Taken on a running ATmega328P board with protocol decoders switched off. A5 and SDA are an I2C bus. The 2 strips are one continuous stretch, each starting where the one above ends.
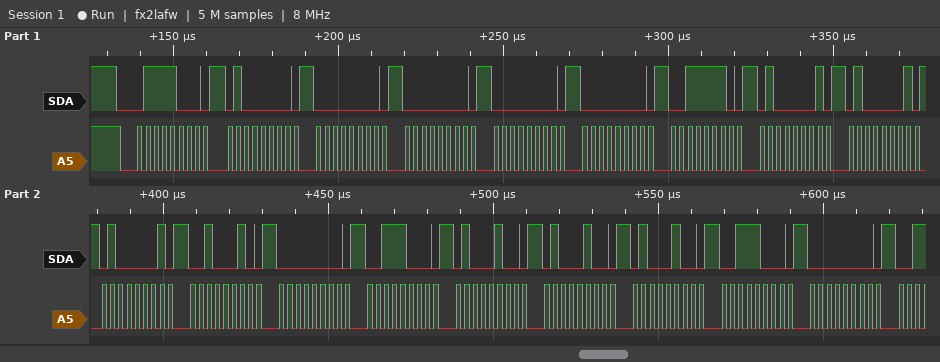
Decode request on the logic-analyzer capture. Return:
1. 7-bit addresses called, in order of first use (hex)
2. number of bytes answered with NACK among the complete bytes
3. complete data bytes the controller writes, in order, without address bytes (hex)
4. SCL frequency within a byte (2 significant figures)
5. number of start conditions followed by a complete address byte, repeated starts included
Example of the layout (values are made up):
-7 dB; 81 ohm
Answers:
0x3C; 0; 40 00 00 00 00 3E 41 41 41 22 00 38 44 44 44 38 00; 400 kHz; 1
